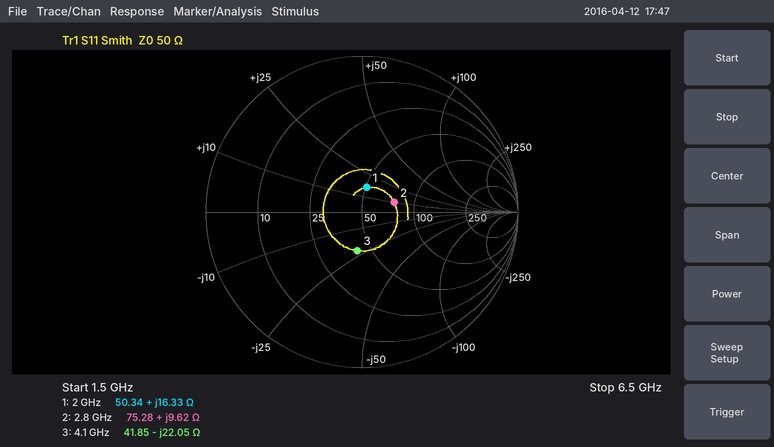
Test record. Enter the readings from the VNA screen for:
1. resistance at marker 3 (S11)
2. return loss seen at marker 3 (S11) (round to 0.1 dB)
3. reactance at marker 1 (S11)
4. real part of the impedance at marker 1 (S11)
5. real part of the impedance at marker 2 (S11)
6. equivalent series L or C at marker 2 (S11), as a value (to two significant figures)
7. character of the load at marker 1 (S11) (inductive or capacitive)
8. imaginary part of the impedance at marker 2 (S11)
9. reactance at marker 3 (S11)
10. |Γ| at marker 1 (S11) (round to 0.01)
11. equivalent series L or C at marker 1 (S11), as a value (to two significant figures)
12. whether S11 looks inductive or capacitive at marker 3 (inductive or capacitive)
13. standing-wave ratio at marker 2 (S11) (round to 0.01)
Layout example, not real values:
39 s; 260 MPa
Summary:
41.85 Ω; 12.1 dB; +16.33 Ω; 50.34 Ω; 75.28 Ω; 550 pH; inductive; +9.62 Ω; -22.05 Ω; 0.16; 1.3 nH; capacitive; 1.55
